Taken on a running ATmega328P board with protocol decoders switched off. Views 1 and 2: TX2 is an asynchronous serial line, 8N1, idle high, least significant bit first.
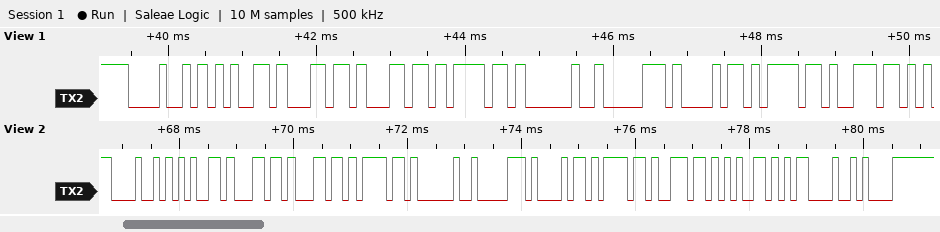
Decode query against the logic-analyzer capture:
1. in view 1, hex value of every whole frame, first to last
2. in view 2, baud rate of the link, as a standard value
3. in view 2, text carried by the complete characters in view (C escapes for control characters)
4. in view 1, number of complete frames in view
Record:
0x48 0x65 0x6C 0x6C 0x6F 0x20 0x70 0x68 0x6F 0x6E
9600 baud
"Hello phone\r\n"
10
